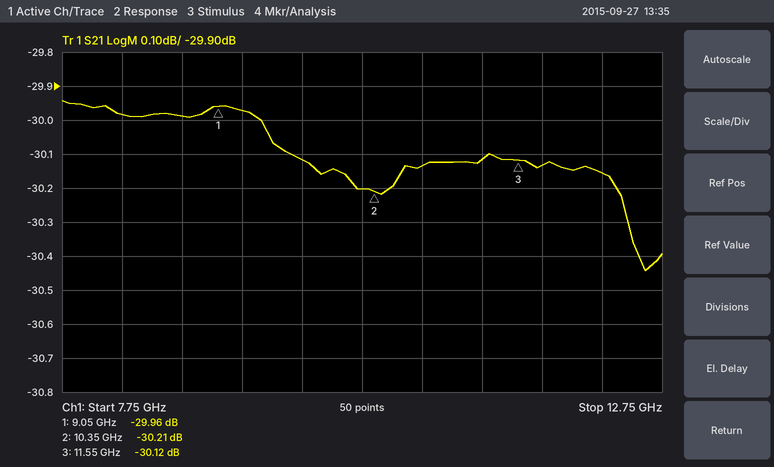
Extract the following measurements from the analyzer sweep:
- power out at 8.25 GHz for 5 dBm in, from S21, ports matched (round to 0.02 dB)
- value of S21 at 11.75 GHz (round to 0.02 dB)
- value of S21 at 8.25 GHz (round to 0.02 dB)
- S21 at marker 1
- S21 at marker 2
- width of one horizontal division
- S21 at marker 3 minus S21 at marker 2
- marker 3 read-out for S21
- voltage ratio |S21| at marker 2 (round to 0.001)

-24.98 dBm
-30.14 dB
-29.98 dB
-29.96 dB
-30.21 dB
500 MHz
0.09 dB
-30.12 dB
0.031
